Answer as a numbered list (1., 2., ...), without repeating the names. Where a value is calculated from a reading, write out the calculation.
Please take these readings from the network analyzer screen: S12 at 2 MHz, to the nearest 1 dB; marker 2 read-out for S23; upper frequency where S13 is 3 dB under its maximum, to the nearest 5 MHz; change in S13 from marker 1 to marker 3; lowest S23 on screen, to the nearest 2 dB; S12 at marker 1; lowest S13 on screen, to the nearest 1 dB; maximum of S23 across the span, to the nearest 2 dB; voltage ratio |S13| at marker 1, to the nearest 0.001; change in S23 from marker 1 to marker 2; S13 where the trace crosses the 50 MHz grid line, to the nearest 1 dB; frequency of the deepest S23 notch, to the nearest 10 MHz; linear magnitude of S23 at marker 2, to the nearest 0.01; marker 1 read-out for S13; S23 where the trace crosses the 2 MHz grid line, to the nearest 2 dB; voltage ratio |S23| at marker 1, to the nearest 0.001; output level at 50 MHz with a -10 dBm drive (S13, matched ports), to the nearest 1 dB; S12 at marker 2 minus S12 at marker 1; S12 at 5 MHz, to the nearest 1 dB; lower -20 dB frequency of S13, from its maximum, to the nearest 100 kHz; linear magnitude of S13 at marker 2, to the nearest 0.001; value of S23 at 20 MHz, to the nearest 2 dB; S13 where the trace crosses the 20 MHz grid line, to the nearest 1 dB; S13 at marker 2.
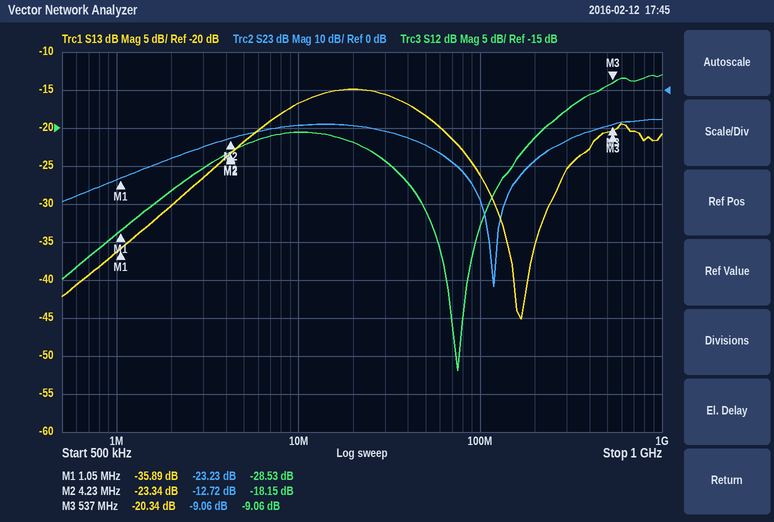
1. -23 dB
2. -12.72 dB
3. 45 MHz
4. -20.34 − (-35.89) = 15.55 dB
5. -52 dB
6. -28.53 dB
7. -45 dB
8. -8 dB
9. 10^(-35.89/20) ≈ 0.016
10. -12.72 − (-23.23) = 10.51 dB
11. -18 dB
12. 120 MHz
13. 10^(-12.72/20) ≈ 0.23
14. -35.89 dB
15. -18 dB
16. 10^(-23.23/20) ≈ 0.069
17. -10 dBm + (-18 dB) = -28 dBm
18. -18.15 − (-28.53) = 10.38 dB
19. -17 dB
20. 1.2 MHz
21. 10^(-23.34/20) ≈ 0.068
22. -10 dB
23. -15 dB
24. -23.34 dB
